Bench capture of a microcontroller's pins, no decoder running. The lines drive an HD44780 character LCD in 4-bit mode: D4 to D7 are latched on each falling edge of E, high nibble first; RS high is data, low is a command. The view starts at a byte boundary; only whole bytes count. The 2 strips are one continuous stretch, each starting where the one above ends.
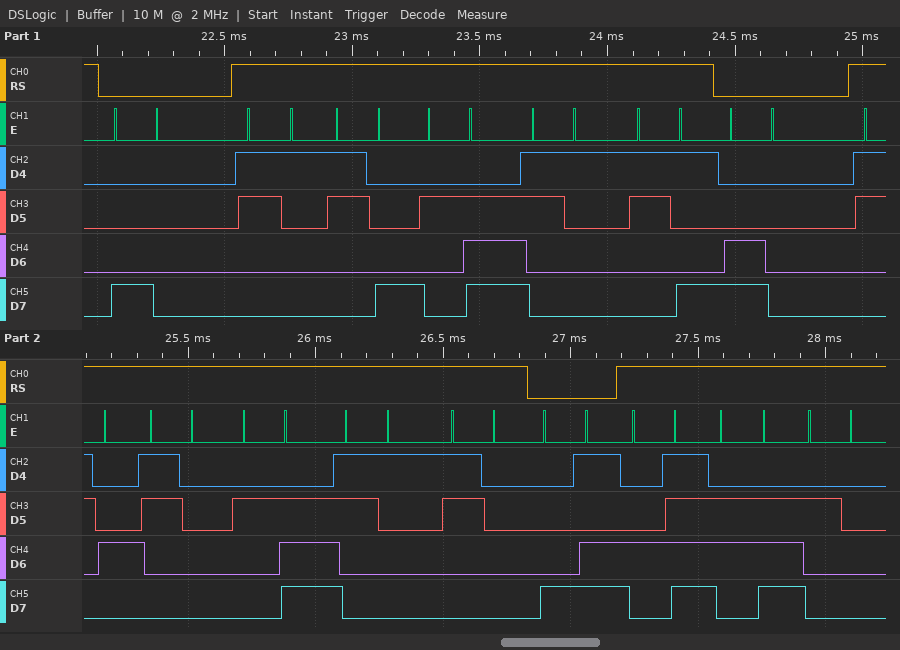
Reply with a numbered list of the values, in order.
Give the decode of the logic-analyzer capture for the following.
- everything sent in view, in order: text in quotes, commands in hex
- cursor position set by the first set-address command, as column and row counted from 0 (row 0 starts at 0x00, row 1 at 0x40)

1. 0x80 "18.19" 0xC0 "40.10" 0x8D "On "
2. column 0, row 0
